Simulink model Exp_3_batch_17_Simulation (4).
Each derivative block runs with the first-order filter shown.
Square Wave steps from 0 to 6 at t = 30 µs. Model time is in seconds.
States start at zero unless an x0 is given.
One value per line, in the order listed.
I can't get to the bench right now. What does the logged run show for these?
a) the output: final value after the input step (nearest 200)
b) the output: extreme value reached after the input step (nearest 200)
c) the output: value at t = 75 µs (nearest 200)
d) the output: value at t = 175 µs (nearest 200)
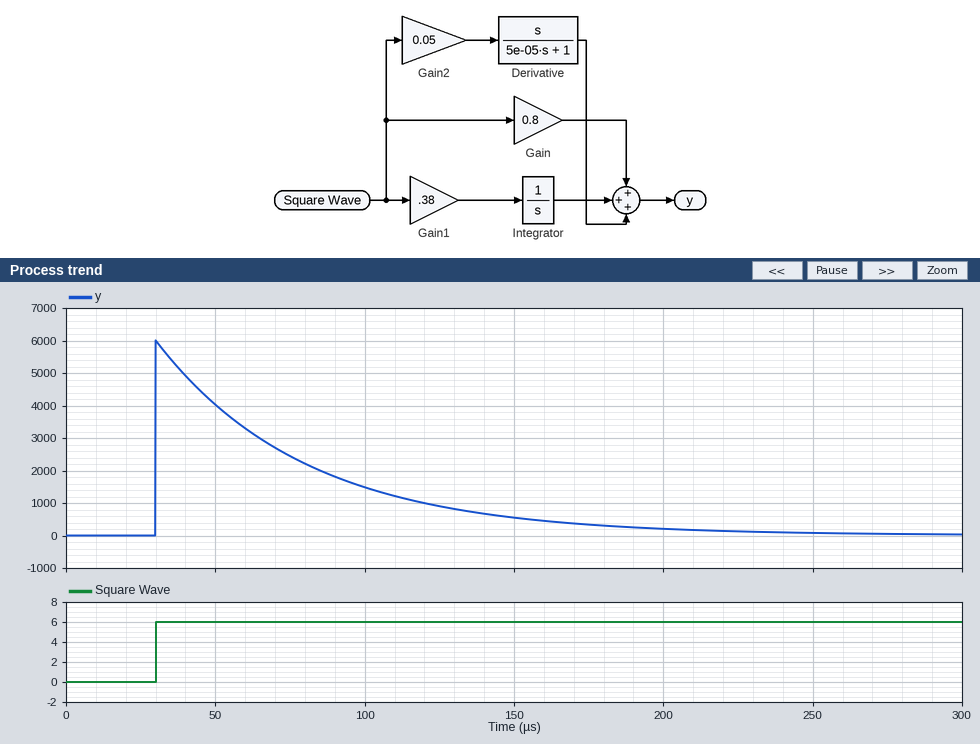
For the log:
0
6000
2400
400
